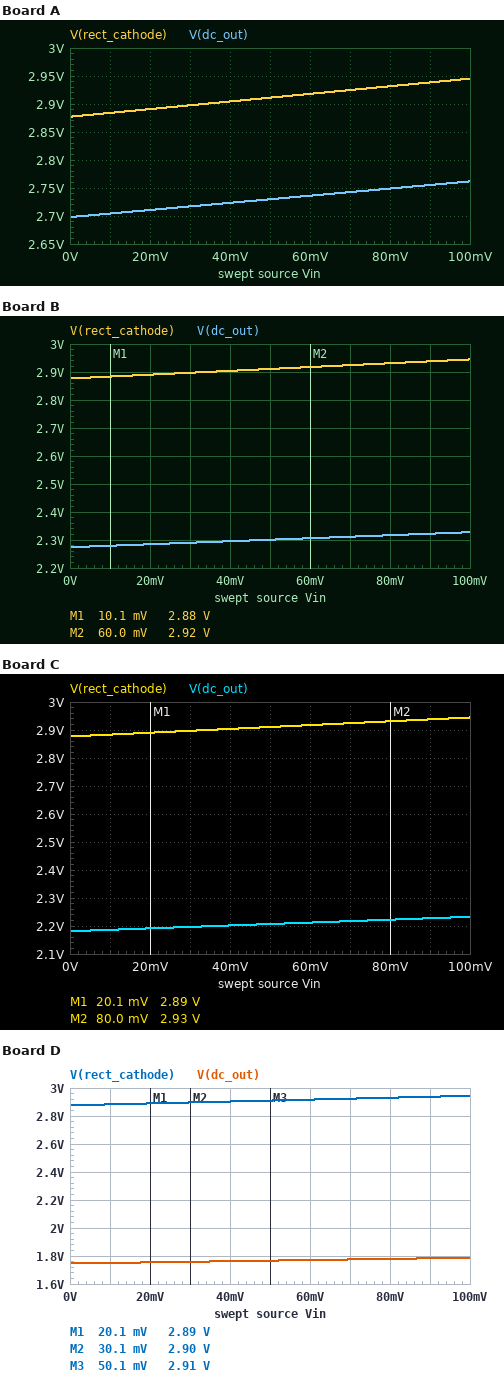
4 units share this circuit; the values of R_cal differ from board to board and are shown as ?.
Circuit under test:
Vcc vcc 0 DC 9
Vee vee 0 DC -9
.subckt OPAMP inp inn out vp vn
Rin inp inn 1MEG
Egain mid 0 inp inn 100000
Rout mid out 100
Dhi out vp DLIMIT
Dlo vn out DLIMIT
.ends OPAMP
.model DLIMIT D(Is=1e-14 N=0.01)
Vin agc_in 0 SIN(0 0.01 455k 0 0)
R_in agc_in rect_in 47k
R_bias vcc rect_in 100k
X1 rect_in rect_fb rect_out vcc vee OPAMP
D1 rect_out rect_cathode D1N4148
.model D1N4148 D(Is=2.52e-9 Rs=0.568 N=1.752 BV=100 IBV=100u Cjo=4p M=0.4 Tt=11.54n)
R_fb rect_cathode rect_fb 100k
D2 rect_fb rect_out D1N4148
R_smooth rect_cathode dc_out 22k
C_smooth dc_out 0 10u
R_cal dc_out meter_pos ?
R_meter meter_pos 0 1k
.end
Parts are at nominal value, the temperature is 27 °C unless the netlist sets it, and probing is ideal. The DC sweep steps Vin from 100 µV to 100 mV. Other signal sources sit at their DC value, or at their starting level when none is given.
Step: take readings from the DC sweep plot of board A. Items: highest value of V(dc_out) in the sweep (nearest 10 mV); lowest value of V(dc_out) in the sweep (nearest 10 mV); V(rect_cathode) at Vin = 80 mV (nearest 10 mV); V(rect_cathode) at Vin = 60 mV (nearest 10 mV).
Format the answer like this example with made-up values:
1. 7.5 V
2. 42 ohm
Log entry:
1. 2.76 V
2. 2.70 V
3. 2.93 V
4. 2.92 V
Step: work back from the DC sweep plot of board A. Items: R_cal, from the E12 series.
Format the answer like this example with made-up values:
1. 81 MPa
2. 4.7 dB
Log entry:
1. 330 kΩ
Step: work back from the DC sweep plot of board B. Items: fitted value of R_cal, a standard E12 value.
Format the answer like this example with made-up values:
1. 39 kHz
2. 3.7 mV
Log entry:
1. 82 kΩ
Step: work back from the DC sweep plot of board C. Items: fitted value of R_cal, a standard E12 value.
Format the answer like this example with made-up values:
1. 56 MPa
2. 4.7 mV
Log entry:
1. 68 kΩ
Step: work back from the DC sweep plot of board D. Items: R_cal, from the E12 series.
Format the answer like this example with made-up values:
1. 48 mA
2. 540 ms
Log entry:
1. 33 kΩ
